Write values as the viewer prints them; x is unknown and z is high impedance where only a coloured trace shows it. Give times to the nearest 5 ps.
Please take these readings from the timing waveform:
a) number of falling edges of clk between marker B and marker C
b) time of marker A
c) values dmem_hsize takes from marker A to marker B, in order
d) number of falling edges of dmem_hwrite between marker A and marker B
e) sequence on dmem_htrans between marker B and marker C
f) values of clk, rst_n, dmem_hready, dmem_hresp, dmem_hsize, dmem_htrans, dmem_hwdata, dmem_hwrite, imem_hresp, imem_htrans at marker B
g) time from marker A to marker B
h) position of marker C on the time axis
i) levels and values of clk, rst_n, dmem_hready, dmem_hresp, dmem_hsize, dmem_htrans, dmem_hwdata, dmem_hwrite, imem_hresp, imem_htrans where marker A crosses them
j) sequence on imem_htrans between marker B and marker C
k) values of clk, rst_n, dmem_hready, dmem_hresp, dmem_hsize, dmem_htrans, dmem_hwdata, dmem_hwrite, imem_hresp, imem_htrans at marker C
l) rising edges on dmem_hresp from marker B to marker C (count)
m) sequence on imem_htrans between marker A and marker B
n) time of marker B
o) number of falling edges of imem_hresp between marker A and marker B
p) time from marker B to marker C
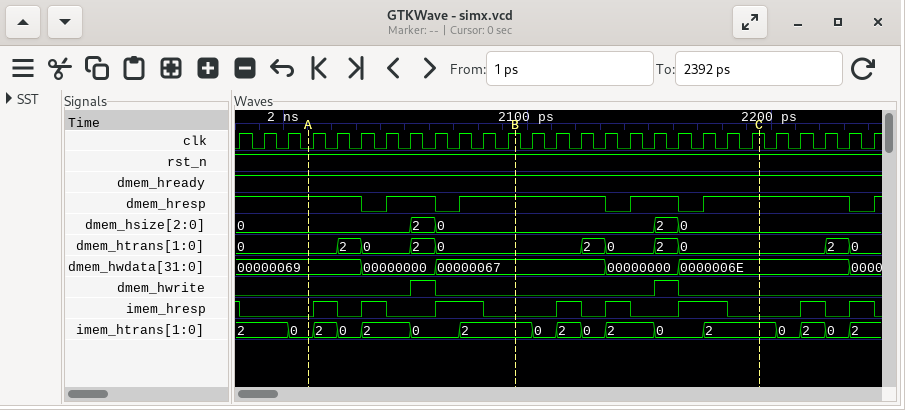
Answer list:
10
2010 ps
0, 2, 0
1
0, 2, 0, 2, 0
clk=1, rst_n=1, dmem_hready=1, dmem_hresp=1, dmem_hsize=0, dmem_htrans=0, dmem_hwdata=00000067, dmem_hwrite=0, imem_hresp=0, imem_htrans=2
85 ps
2195 ps
clk=0, rst_n=1, dmem_hready=1, dmem_hresp=1, dmem_hsize=0, dmem_htrans=0, dmem_hwdata=00000069, dmem_hwrite=0, imem_hresp=0, imem_htrans=0
2, 0, 2, 0, 2, 0, 2
clk=1, rst_n=1, dmem_hready=1, dmem_hresp=1, dmem_hsize=0, dmem_htrans=0, dmem_hwdata=0000006E, dmem_hwrite=0, imem_hresp=0, imem_htrans=2
2
0, 2, 0, 2, 0, 2
2095 ps
3
100 ps
